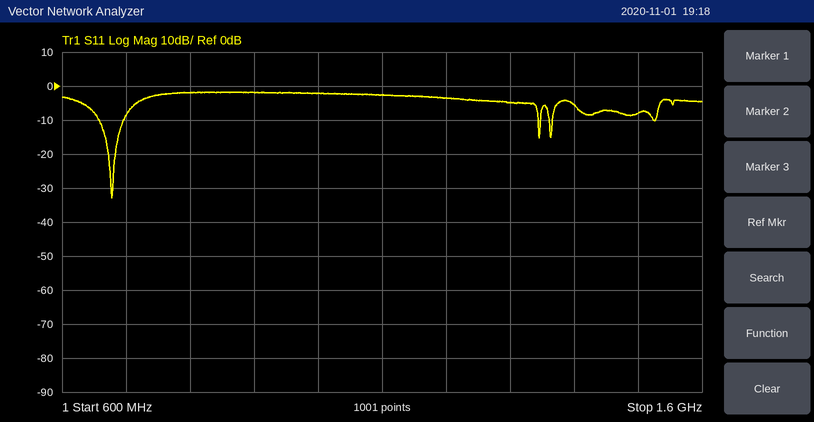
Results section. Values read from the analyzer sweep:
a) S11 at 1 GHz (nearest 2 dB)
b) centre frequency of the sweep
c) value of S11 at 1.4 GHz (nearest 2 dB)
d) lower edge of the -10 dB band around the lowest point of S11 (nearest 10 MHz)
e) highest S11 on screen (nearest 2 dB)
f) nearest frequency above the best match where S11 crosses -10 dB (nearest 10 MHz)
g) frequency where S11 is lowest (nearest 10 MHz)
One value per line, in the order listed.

-2 dB
1.1 GHz
-6 dB
660 MHz
-2 dB
700 MHz
680 MHz
